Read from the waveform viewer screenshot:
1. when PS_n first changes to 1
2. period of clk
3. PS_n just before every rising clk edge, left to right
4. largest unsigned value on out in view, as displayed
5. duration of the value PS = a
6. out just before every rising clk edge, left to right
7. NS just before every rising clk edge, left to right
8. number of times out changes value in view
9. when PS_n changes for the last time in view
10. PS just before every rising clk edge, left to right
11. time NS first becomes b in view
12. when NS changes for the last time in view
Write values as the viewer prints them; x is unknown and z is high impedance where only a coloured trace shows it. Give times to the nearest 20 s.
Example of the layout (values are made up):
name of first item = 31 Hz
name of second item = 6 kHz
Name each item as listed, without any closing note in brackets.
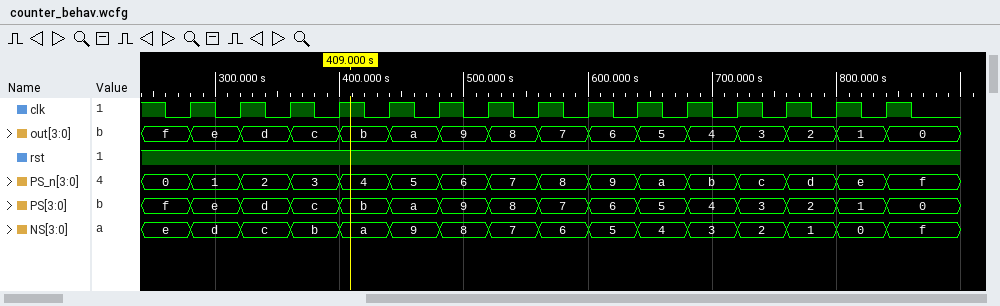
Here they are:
when PS_n first changes to 1 = 280 s
period of clk = 40 s
PS_n just before every rising clk edge, left to right = 0, 1, 2, 3, 4, 5, 6, 7, 8, 9, a, b, c, d, e
largest unsigned value on out in view, as displayed = f
duration of the value PS = a = 40 s
out just before every rising clk edge, left to right = f, e, d, c, b, a, 9, 8, 7, 6, 5, 4, 3, 2, 1
NS just before every rising clk edge, left to right = e, d, c, b, a, 9, 8, 7, 6, 5, 4, 3, 2, 1, 0
number of times out changes value in view = 15
when PS_n changes for the last time in view = 840 s
PS just before every rising clk edge, left to right = f, e, d, c, b, a, 9, 8, 7, 6, 5, 4, 3, 2, 1
time NS first becomes b in view = 360 s
when NS changes for the last time in view = 840 s
